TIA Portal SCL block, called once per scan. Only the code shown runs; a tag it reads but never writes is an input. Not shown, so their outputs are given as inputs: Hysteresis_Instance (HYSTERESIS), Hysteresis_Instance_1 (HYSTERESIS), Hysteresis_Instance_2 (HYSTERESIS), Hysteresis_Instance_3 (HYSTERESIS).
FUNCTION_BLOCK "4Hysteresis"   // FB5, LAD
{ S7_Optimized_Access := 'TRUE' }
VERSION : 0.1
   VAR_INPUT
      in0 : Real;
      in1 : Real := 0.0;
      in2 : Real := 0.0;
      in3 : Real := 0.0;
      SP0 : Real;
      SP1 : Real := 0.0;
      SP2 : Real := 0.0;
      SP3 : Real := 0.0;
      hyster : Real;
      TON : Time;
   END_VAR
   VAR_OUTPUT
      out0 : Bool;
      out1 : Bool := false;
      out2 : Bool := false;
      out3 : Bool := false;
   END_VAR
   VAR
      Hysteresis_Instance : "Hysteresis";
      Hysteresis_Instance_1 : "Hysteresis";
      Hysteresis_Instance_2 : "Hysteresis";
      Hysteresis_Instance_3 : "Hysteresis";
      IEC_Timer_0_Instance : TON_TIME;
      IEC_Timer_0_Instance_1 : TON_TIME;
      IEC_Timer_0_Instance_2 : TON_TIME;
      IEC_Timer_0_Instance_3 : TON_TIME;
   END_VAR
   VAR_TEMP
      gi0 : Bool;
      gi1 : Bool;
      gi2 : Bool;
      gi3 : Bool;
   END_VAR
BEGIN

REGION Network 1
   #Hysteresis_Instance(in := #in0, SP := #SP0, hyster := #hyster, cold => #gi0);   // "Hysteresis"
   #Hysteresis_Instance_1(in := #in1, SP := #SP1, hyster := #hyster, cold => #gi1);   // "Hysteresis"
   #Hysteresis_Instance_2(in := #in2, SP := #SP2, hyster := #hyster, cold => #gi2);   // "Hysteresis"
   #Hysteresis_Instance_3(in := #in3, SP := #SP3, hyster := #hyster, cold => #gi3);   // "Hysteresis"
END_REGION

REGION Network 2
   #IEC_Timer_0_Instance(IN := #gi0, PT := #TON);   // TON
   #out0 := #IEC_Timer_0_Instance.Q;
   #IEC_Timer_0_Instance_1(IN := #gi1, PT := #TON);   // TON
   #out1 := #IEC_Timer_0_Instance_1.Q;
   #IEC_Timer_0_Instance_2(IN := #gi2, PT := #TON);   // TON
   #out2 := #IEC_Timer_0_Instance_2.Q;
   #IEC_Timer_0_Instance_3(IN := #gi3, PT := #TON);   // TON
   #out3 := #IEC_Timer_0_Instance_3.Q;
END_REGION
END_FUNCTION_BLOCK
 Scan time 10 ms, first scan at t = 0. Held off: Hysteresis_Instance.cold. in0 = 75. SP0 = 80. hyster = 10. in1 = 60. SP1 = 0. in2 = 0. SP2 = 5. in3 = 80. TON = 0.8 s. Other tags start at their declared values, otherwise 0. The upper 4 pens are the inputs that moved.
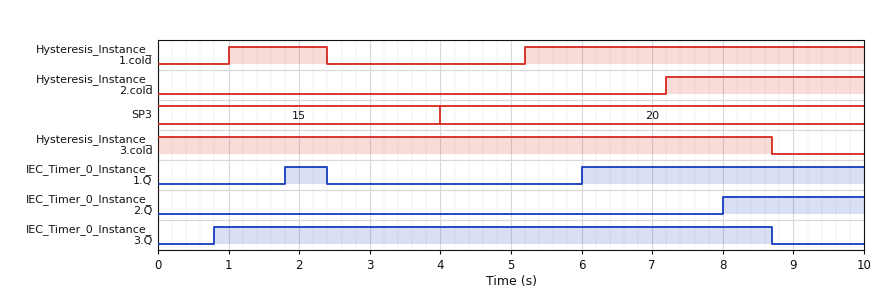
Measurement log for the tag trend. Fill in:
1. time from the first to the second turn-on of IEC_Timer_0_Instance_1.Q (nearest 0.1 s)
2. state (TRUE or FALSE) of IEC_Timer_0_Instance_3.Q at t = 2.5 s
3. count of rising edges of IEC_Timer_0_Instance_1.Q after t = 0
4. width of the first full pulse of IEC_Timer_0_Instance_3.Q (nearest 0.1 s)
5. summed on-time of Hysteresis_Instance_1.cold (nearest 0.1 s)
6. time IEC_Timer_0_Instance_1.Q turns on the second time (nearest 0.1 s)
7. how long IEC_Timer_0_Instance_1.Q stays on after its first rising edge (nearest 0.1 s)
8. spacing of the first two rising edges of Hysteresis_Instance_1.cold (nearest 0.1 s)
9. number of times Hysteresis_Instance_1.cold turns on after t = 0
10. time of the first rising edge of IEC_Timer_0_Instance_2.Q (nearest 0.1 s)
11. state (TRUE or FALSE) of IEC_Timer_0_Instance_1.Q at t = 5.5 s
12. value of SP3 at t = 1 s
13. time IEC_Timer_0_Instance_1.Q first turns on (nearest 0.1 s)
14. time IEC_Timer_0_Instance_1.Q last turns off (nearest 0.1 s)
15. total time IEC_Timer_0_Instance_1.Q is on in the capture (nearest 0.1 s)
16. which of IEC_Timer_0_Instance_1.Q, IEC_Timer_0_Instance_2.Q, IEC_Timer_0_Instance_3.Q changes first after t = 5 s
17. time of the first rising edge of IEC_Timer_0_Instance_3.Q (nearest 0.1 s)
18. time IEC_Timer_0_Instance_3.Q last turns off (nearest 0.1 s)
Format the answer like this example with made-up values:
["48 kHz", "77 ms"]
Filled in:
["4.2 s", "TRUE", "2", "7.9 s", "6.2 s", "6.0 s", "0.6 s", "4.2 s", "2", "8.0 s", "FALSE", "15", "1.8 s", "2.4 s", "4.6 s", "IEC_Timer_0_Instance_1.Q", "0.8 s", "8.7 s"]
